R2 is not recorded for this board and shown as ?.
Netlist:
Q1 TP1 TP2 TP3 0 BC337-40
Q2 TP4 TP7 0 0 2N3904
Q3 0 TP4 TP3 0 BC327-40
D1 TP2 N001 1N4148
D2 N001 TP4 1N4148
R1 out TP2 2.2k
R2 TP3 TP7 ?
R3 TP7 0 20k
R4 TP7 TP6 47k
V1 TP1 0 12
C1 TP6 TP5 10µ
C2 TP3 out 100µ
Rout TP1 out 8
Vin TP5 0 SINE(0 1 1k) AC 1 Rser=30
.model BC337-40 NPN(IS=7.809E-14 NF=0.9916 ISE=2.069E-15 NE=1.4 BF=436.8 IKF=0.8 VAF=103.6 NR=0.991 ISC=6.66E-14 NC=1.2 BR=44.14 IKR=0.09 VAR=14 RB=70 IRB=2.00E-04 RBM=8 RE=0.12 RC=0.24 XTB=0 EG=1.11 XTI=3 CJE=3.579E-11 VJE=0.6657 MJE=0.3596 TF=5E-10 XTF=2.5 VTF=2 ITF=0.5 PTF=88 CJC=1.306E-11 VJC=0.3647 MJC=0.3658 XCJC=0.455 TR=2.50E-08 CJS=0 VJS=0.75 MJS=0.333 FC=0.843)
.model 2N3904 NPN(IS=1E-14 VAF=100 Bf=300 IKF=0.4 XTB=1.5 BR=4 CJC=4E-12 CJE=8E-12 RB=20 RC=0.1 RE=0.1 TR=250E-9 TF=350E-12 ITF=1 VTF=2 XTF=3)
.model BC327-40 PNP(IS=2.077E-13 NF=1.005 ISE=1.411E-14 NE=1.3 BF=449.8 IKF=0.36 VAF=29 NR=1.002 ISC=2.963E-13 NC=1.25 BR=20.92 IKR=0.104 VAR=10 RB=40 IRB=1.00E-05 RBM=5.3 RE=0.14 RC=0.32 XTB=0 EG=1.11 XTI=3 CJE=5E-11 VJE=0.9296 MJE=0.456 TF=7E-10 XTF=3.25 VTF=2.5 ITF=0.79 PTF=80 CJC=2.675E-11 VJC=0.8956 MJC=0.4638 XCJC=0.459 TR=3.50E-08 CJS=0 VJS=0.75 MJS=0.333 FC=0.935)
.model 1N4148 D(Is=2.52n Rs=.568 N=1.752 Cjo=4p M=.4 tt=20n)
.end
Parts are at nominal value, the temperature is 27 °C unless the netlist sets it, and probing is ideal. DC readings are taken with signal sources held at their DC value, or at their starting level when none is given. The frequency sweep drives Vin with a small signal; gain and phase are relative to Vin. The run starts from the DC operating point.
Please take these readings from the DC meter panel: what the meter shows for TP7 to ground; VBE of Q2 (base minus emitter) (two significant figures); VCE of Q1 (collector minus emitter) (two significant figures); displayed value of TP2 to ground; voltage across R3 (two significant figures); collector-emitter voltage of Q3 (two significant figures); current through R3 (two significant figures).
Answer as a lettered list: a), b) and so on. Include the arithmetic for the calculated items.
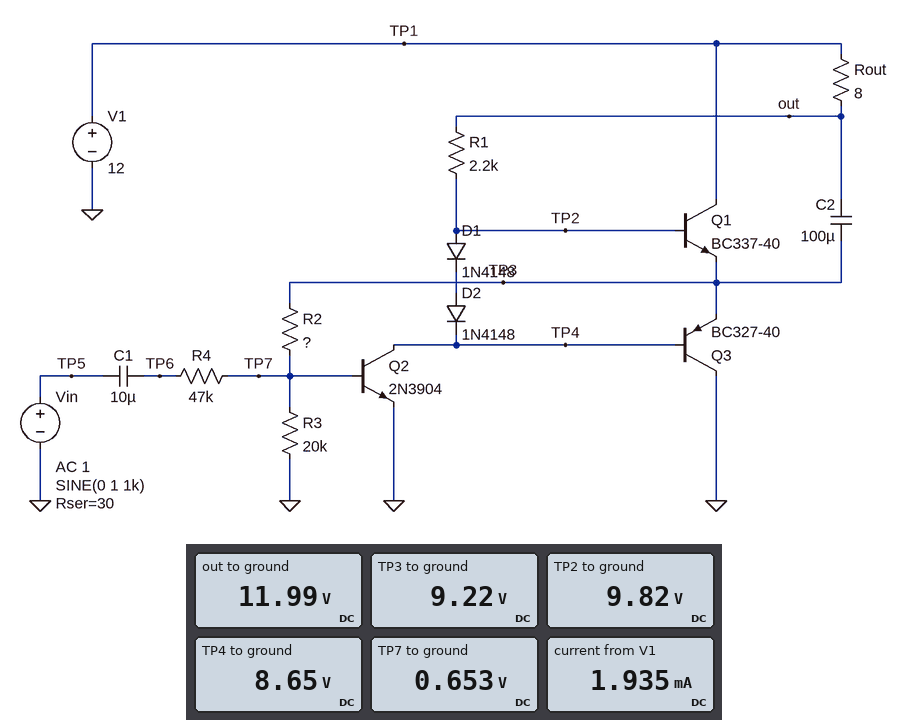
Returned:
a) 0.653 V
b) 653 mV = 650 mV
c) 12 V - 9.22 V = 2.8 V
d) 9.82 V
e) 653 mV = 650 mV
f) 0 V - 9.22 V = -9.2 V
g) (653 mV) / 20 kΩ = 33 µA
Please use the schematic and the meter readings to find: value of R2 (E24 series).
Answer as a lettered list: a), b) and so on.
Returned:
a) 240 kΩ
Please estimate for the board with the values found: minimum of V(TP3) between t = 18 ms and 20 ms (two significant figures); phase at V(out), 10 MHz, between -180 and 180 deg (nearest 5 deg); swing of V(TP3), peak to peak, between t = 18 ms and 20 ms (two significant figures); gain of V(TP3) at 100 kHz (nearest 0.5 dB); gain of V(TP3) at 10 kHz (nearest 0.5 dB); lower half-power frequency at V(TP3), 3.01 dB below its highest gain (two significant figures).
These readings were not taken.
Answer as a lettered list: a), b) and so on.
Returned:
a) 6.0 V
b) 30 deg
c) 5.4 V
d) 6.0 dB
e) 7.0 dB
f) 320 mHz
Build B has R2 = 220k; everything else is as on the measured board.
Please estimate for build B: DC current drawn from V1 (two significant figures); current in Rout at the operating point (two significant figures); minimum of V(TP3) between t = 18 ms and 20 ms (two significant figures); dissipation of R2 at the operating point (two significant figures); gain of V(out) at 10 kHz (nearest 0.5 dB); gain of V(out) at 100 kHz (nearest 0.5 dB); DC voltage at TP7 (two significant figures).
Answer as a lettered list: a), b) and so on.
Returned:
a) 2.5 mA
b) 1.2 mA
c) 5.6 V
d) 300 µW
e) 8.0 dB
f) 7.0 dB
g) 660 mV
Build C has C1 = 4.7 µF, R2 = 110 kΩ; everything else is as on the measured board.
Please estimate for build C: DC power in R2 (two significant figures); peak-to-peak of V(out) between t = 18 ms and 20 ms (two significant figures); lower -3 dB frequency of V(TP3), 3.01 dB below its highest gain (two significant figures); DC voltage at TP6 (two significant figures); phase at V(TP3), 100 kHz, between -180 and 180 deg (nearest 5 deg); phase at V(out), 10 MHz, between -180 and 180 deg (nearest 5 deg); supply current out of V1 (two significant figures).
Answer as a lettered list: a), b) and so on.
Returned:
a) 200 µW
b) 3.8 V
c) 720 mHz
d) 680 mV
e) 170 deg
f) 35 deg
g) 7.9 mA
